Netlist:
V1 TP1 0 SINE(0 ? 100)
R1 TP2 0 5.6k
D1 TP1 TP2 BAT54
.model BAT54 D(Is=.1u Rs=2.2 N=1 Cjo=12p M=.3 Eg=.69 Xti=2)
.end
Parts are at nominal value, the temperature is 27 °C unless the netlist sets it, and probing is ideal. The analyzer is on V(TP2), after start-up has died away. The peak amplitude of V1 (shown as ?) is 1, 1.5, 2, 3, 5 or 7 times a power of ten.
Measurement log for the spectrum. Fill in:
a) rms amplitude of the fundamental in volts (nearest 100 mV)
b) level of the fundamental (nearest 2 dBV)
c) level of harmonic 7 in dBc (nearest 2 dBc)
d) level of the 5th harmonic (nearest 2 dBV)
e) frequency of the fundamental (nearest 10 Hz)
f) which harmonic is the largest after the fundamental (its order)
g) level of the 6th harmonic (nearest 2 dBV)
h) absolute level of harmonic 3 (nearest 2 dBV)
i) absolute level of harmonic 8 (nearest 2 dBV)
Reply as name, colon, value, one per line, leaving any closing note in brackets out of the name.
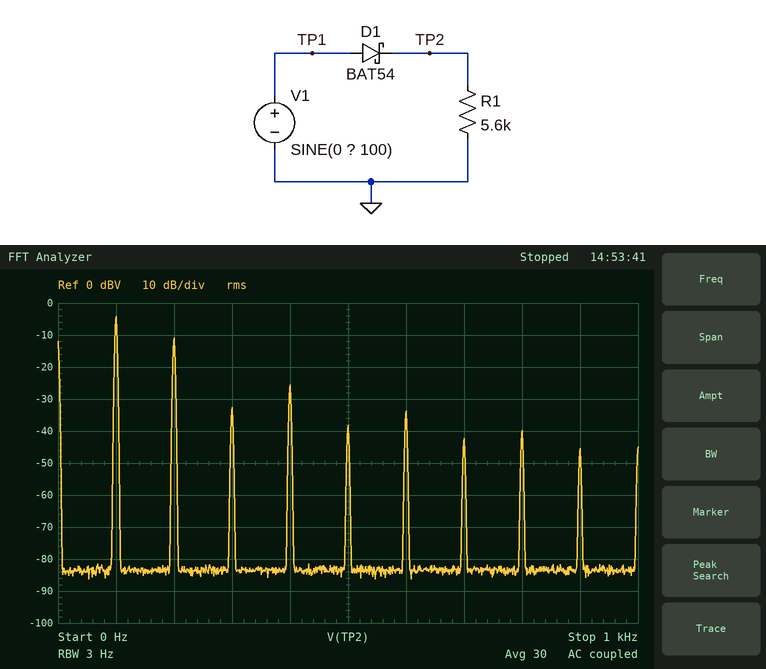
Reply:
rms amplitude of the fundamental in volts: 600 mV
level of the fundamental: -4 dBV
level of harmonic 7 in dBc: -38 dBc
level of the 5th harmonic: -38 dBV
frequency of the fundamental: 100 Hz
which harmonic is the largest after the fundamental: 2
level of the 6th harmonic: -34 dBV
absolute level of harmonic 3: -32 dBV
absolute level of harmonic 8: -40 dBV
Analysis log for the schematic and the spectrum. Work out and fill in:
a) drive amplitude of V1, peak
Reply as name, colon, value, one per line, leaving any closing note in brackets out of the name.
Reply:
drive amplitude of V1, peak: 2 V
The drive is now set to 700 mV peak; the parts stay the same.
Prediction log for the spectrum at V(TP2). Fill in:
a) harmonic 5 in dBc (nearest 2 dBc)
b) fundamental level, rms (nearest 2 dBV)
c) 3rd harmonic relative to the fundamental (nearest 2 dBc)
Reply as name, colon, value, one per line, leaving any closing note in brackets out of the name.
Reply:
harmonic 5 in dBc: -28 dBc
fundamental level, rms: -16 dBV
3rd harmonic relative to the fundamental: -20 dBc
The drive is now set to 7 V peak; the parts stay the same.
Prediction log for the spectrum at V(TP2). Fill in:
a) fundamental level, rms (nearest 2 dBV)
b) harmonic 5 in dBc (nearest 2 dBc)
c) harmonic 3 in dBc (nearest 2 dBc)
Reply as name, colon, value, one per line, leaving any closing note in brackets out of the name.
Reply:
fundamental level, rms: 8 dBV
harmonic 5 in dBc: -44 dBc
harmonic 3 in dBc: -38 dBc
